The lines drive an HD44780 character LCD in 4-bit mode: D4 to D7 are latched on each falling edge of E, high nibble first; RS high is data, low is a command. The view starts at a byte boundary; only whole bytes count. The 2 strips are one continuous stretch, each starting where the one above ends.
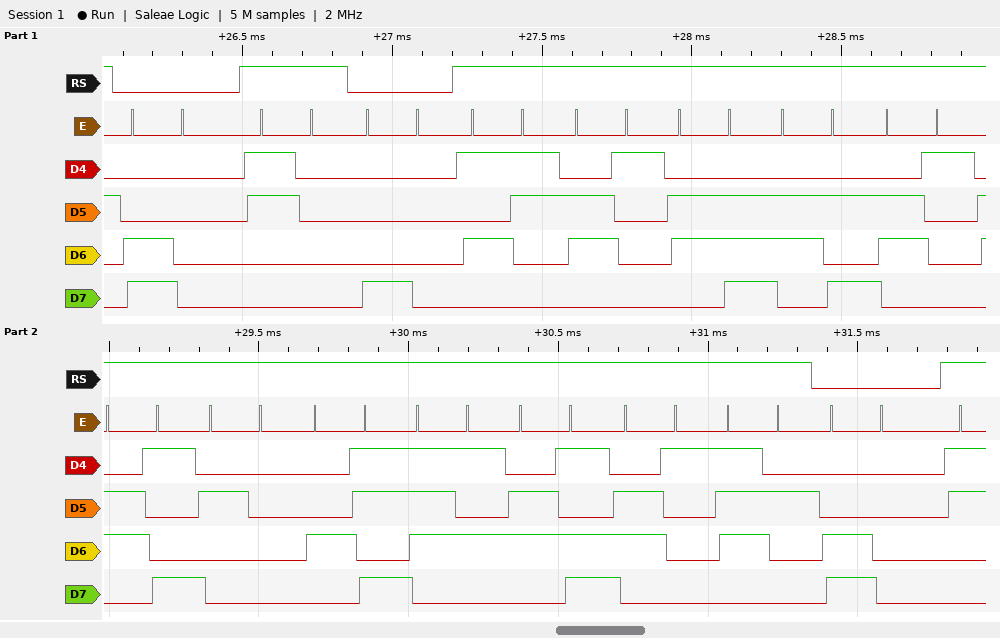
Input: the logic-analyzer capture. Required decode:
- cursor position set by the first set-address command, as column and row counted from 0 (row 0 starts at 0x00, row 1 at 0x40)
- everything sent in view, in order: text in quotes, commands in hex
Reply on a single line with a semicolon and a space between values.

column 0, row 1; 0xC0 "0" 0x80 "Sanjai Kumar" 0xC0
